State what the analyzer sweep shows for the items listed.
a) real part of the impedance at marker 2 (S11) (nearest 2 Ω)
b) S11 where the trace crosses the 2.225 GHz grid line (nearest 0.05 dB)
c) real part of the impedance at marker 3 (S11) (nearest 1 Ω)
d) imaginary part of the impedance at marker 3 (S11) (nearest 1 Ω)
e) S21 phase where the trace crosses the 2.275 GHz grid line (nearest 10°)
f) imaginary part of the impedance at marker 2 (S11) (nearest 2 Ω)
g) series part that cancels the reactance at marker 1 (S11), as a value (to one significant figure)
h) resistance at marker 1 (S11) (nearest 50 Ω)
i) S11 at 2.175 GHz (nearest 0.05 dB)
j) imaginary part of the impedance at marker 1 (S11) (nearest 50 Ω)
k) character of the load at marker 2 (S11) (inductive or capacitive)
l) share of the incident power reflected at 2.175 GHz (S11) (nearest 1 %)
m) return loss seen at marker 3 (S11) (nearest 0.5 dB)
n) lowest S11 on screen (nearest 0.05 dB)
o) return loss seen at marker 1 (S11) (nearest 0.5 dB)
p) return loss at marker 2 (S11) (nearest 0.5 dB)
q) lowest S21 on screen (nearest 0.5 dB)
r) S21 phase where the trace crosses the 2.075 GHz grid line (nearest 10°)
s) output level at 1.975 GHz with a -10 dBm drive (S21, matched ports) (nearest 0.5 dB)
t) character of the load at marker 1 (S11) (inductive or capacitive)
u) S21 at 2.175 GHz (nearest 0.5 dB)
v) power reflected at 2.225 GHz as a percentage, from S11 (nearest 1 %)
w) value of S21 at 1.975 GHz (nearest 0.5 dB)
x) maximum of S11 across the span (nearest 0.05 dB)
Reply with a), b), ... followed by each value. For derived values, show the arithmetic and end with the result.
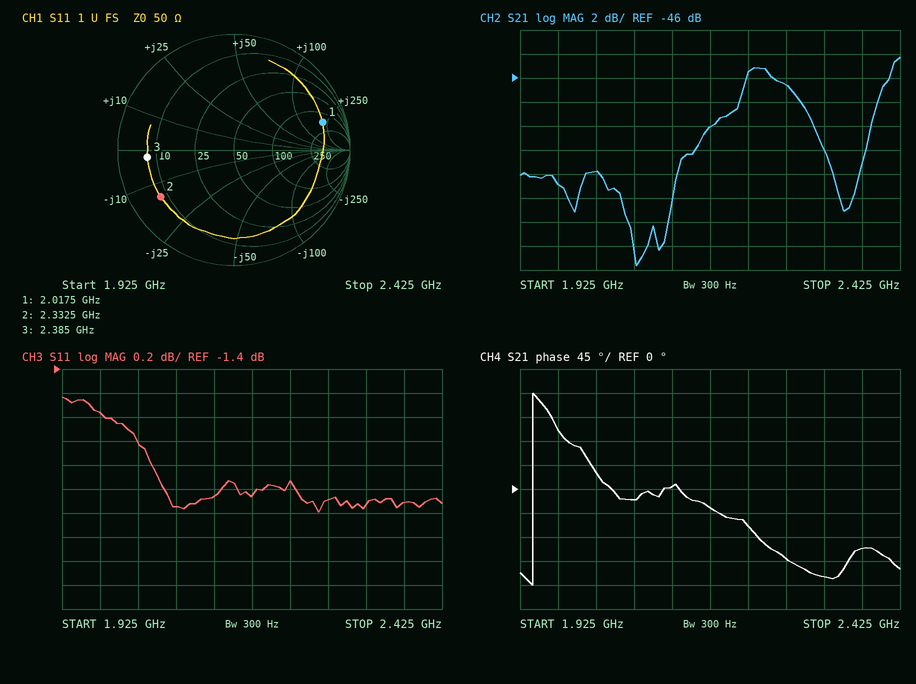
a) 8 Ω
b) -2.35 dB
c) 7 Ω
d) -2 Ω
e) -130°
f) -14 Ω
g) C = 1/(2π × 2.0175 GHz × 200 Ω) ≈ 394 fF, so 400 fF to one significant figure
h) 150 Ω
i) -2.45 dB
j) +200 Ω
k) capacitive
l) 10^(-2.45/10) ≈ 57 %
m) 2.5 dB
n) -2.60 dB
o) 2.0 dB
p) 2.5 dB
q) -61.5 dB
r) -20°
s) -10 dBm + (-55.0 dB) = -65.0 dBm
t) inductive
u) -50.0 dB
v) 10^(-2.35/10) ≈ 58 %
w) -55.0 dB
x) -1.65 dB
